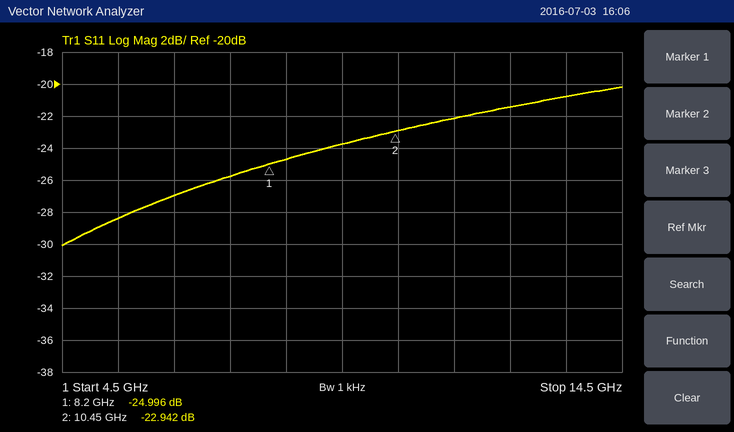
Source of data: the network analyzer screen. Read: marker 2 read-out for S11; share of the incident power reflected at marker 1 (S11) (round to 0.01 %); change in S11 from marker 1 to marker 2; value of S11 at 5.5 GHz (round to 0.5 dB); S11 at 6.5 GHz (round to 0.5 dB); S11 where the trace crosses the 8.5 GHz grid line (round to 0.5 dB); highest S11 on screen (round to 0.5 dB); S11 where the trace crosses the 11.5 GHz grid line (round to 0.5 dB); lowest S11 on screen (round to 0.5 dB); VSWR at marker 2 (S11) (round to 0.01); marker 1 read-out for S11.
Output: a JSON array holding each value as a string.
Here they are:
["-22.942 dB", "0.32 %", "2.054 dB", "-28.5 dB", "-27.0 dB", "-24.5 dB", "-20.0 dB", "-22.0 dB", "-30.0 dB", "1.15", "-24.996 dB"]
